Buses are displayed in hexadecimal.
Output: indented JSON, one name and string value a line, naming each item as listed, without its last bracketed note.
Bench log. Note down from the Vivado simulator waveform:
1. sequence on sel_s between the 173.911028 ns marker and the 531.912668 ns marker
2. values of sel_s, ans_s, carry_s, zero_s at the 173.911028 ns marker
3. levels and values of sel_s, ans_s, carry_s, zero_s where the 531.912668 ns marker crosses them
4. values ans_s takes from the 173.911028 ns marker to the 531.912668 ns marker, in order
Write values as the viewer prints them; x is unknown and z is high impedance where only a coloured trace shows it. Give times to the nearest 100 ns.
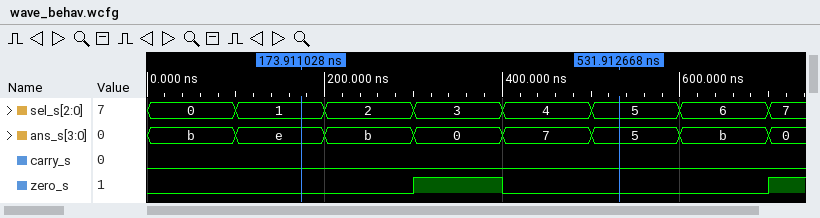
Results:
{
  "sequence on sel_s between the 173.911028 ns marker and the 531.912668 ns marker": "1, 2, 3, 4, 5",
  "values of sel_s, ans_s, carry_s, zero_s at the 173.911028 ns marker": "sel_s=1, ans_s=e, carry_s=0, zero_s=0",
  "levels and values of sel_s, ans_s, carry_s, zero_s where the 531.912668 ns marker crosses them": "sel_s=5, ans_s=5, carry_s=0, zero_s=0",
  "values ans_s takes from the 173.911028 ns marker to the 531.912668 ns marker, in order": "e, b, 0, 7, 5"
}
